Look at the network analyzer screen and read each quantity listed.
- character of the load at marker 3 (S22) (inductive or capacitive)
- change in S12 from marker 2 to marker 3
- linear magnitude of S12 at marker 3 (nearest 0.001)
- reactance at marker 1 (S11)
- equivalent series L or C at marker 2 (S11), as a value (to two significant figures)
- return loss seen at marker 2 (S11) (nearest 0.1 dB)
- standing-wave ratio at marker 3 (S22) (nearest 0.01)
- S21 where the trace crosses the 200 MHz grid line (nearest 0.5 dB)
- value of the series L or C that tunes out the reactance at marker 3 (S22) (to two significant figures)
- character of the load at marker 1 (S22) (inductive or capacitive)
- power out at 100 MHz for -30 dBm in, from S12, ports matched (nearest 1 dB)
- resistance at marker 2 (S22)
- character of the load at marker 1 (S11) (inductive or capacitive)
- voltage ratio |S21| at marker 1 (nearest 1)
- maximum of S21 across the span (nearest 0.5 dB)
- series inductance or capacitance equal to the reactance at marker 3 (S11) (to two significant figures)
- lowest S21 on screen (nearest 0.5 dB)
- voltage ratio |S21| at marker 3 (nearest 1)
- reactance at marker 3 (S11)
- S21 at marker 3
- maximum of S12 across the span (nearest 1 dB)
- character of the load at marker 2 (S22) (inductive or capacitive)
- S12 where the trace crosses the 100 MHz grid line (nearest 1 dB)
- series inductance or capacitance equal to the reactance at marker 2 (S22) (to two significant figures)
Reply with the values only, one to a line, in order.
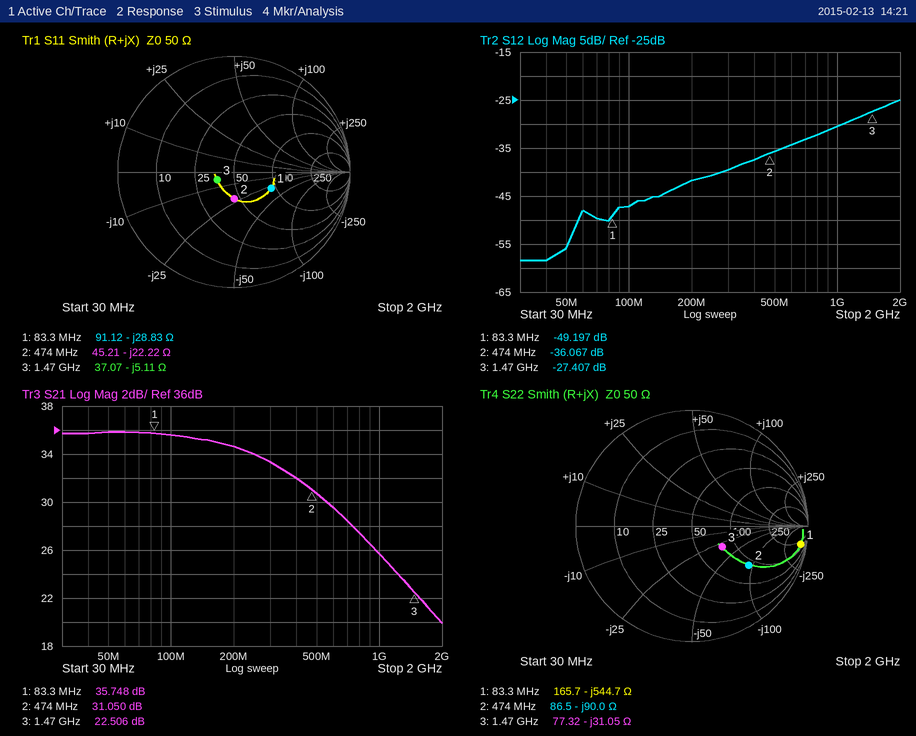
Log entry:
capacitive
8.660 dB
0.043
-28.83 Ω
15 pF
12.7 dB
1.92
34.5 dB
3.4 nH
capacitive
-77 dBm
86.5 Ω
capacitive
61
36.0 dB
21 pF
20.0 dB
13
-5.11 Ω
22.506 dB
-25 dB
capacitive
-47 dB
3.7 pF
